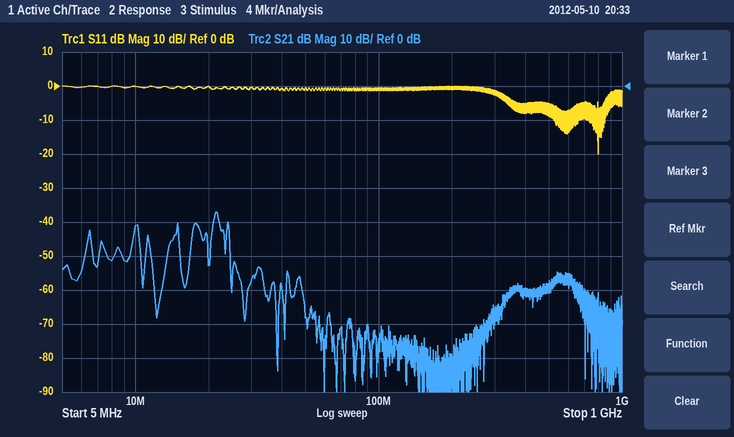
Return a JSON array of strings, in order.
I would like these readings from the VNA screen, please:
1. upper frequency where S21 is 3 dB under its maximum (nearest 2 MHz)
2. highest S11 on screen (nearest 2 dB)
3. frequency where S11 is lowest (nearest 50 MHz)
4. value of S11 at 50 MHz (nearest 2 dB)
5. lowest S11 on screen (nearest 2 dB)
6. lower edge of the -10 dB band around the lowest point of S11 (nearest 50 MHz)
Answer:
["22 MHz", "0 dB", "800 MHz", "0 dB", "-20 dB", "800 MHz"]
